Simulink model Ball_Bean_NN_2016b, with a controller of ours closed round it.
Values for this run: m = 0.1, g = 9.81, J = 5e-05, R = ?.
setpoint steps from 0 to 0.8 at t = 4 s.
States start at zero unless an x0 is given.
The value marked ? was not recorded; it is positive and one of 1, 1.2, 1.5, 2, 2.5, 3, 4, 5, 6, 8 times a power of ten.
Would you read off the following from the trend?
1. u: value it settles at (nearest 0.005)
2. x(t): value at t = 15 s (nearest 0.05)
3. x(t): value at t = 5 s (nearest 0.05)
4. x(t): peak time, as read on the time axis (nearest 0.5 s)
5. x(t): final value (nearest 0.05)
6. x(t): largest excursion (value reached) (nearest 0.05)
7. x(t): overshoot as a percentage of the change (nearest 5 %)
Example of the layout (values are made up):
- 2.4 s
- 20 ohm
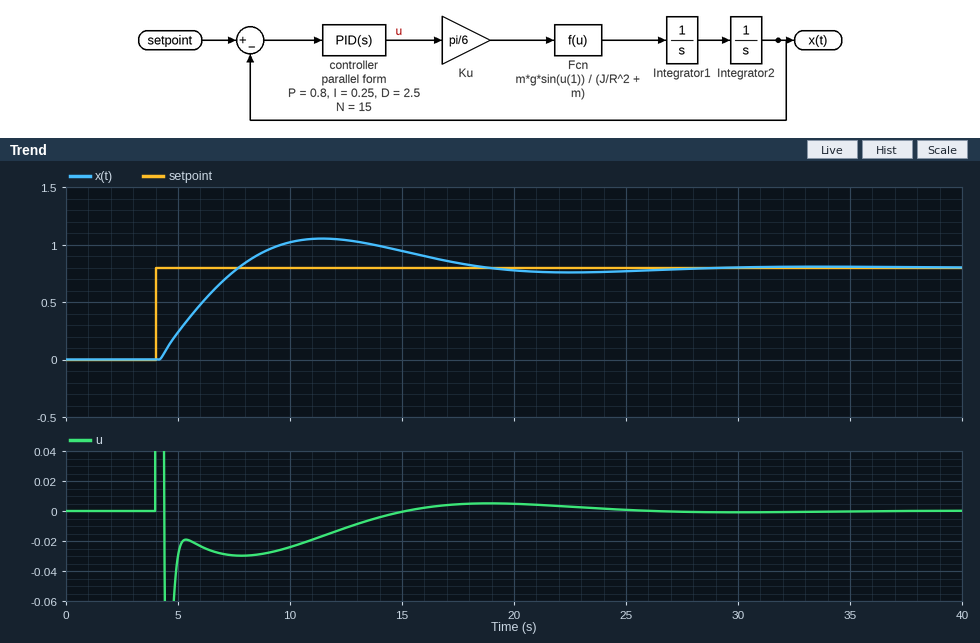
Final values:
- 0.000
- 0.95
- 0.25
- 11.5 s
- 0.80
- 1.05
- 30 %
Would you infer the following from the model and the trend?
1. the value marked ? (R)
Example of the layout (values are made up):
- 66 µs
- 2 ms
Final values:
- 0.015
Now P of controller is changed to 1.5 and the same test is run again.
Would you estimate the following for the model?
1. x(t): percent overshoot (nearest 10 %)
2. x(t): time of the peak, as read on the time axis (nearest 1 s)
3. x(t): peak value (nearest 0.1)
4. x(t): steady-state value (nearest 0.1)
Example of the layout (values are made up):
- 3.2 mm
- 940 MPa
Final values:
- 20 %
- 10 s
- 0.9
- 0.8
